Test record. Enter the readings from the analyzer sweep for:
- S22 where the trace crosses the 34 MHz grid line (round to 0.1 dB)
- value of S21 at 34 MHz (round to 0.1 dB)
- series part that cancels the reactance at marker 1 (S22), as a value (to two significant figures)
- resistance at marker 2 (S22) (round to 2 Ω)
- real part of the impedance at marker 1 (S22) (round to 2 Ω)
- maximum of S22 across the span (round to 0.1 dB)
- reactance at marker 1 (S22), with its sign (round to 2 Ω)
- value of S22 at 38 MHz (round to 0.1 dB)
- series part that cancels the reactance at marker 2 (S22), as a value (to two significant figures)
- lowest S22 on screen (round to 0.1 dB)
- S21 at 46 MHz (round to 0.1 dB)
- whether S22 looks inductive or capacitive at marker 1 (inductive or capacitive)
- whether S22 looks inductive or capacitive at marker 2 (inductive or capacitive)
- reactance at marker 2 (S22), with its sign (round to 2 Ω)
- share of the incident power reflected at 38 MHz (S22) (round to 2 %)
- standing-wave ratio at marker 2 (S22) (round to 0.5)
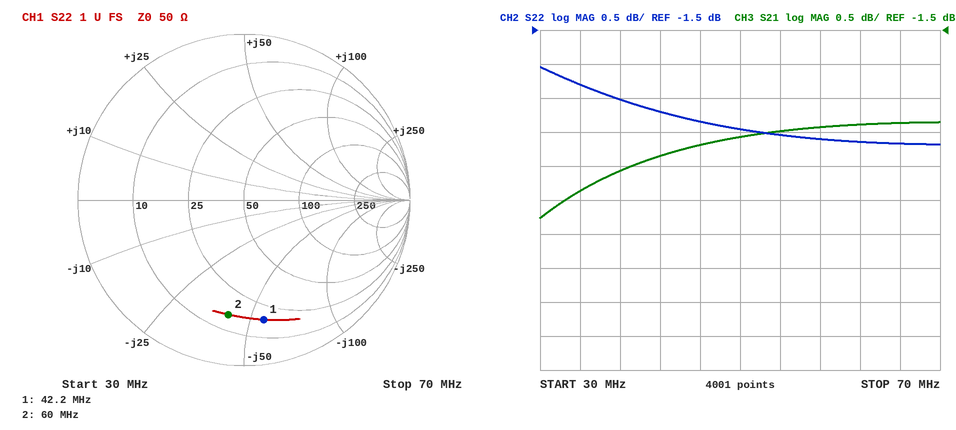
-2.3 dB
-3.9 dB
210 nH
16 Ω
18 Ω
-2.0 dB
-56 Ω
-2.5 dB
110 nH
-3.2 dB
-3.2 dB
capacitive
capacitive
-42 Ω
56 %
5.5
